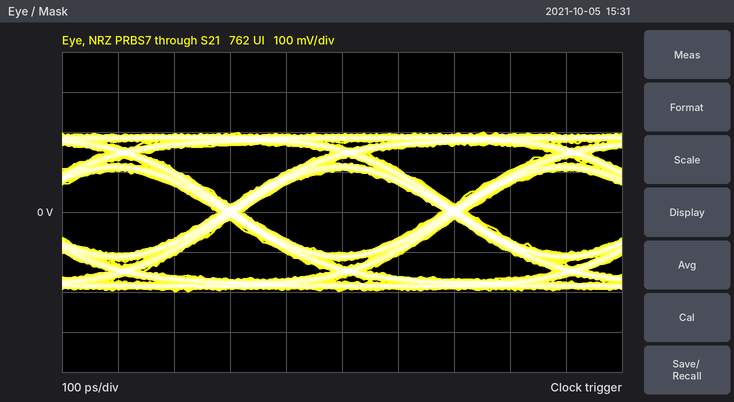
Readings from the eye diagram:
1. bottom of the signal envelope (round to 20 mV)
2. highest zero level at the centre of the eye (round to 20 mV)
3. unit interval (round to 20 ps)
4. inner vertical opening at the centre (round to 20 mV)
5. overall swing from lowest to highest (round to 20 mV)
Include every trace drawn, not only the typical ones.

-200 mV
-100 mV
400 ps
200 mV
400 mV
